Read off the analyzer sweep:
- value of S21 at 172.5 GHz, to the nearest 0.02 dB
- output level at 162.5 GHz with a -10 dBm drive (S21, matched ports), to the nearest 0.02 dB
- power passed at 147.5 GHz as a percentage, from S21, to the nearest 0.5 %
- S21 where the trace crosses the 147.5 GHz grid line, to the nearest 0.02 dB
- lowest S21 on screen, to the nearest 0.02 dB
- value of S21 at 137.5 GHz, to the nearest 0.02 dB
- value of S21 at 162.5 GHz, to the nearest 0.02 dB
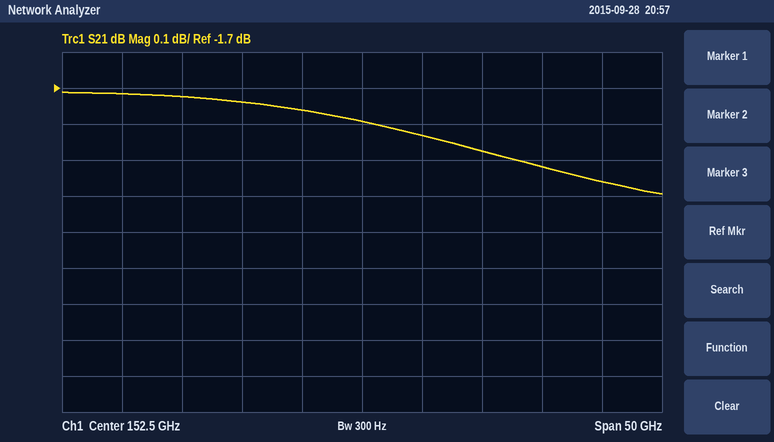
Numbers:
-1.96 dB
-11.88 dBm
66.5 %
-1.76 dB
-2.00 dB
-1.72 dB
-1.88 dB
